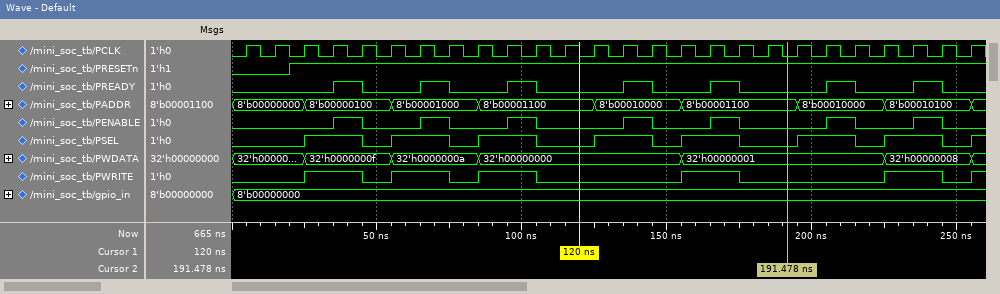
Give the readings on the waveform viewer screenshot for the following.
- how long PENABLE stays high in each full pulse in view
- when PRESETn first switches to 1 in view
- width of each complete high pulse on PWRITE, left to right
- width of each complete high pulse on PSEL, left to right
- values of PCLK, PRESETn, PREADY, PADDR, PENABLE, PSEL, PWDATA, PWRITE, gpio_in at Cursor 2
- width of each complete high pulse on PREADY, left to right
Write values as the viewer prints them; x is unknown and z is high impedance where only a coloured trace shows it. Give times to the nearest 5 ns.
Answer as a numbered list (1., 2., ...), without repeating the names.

1. 10 ns, 10 ns, 10 ns, 10 ns, 10 ns, 10 ns, 10 ns
2. 20 ns
3. 20 ns, 20 ns, 20 ns, 20 ns, 20 ns
4. 20 ns, 20 ns, 20 ns, 20 ns, 20 ns, 20 ns, 20 ns
5. PCLK=0, PRESETn=1, PREADY=0, PADDR=8'b00001100, PENABLE=0, PSEL=0, PWDATA=32'h00000001, PWRITE=0, gpio_in=8'b00000000
6. 10 ns, 10 ns, 10 ns, 10 ns, 10 ns, 10 ns, 10 ns
